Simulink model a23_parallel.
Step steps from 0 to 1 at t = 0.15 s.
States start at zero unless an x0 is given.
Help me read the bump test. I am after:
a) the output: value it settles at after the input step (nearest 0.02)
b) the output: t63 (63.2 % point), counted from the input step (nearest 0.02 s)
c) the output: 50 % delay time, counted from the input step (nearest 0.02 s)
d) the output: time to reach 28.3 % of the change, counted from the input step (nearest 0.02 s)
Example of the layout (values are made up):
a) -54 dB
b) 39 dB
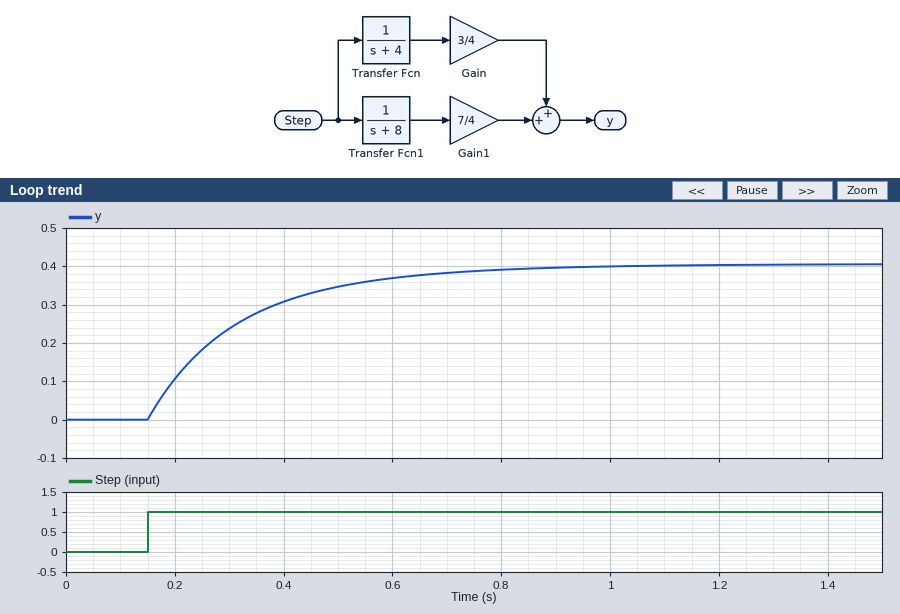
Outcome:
a) 0.40
b) 0.18 s
c) 0.12 s
d) 0.06 s
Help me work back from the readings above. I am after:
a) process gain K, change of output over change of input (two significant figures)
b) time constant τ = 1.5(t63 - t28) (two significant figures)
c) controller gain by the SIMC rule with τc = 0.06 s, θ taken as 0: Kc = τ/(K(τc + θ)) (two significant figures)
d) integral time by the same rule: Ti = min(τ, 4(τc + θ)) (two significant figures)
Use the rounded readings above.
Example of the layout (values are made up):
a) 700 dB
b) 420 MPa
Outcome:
a) 0.40
b) 0.18 s
c) 7.5
d) 0.18 s
